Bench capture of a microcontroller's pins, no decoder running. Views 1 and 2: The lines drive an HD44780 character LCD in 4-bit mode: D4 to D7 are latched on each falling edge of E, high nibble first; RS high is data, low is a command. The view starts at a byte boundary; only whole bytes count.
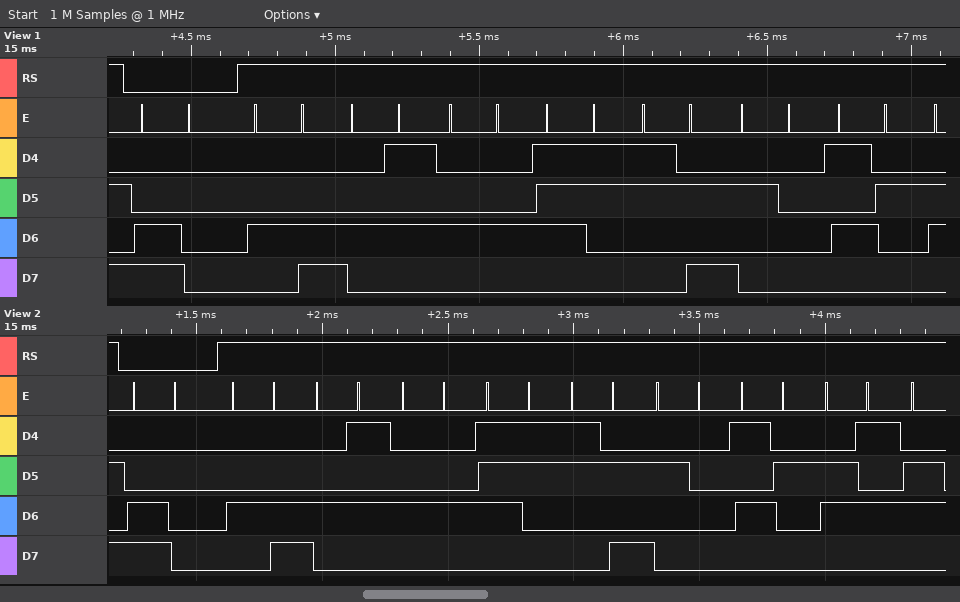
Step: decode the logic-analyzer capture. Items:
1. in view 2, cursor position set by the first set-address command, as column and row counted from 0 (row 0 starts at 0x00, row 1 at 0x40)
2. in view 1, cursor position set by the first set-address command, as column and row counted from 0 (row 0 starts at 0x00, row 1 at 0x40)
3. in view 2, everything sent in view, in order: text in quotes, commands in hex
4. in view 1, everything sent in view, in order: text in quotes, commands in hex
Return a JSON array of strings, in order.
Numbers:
["column 0, row 1", "column 0, row 1", "0xC0 \"LEDs: Re\"", "0xC0 \"LEDs: R\""]
